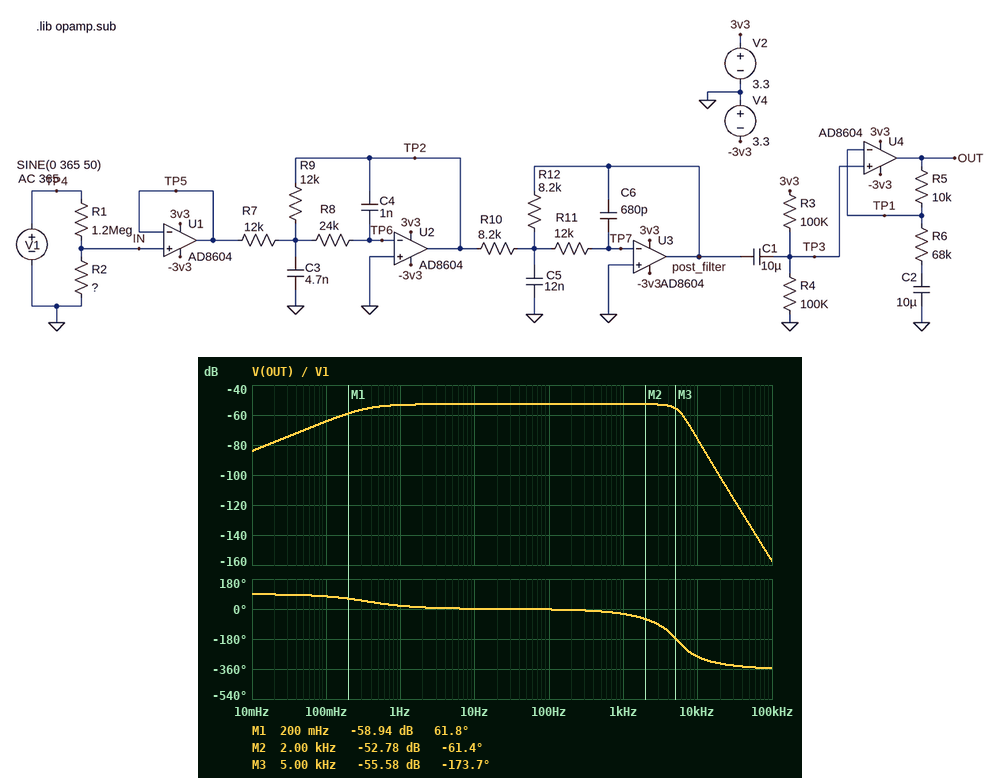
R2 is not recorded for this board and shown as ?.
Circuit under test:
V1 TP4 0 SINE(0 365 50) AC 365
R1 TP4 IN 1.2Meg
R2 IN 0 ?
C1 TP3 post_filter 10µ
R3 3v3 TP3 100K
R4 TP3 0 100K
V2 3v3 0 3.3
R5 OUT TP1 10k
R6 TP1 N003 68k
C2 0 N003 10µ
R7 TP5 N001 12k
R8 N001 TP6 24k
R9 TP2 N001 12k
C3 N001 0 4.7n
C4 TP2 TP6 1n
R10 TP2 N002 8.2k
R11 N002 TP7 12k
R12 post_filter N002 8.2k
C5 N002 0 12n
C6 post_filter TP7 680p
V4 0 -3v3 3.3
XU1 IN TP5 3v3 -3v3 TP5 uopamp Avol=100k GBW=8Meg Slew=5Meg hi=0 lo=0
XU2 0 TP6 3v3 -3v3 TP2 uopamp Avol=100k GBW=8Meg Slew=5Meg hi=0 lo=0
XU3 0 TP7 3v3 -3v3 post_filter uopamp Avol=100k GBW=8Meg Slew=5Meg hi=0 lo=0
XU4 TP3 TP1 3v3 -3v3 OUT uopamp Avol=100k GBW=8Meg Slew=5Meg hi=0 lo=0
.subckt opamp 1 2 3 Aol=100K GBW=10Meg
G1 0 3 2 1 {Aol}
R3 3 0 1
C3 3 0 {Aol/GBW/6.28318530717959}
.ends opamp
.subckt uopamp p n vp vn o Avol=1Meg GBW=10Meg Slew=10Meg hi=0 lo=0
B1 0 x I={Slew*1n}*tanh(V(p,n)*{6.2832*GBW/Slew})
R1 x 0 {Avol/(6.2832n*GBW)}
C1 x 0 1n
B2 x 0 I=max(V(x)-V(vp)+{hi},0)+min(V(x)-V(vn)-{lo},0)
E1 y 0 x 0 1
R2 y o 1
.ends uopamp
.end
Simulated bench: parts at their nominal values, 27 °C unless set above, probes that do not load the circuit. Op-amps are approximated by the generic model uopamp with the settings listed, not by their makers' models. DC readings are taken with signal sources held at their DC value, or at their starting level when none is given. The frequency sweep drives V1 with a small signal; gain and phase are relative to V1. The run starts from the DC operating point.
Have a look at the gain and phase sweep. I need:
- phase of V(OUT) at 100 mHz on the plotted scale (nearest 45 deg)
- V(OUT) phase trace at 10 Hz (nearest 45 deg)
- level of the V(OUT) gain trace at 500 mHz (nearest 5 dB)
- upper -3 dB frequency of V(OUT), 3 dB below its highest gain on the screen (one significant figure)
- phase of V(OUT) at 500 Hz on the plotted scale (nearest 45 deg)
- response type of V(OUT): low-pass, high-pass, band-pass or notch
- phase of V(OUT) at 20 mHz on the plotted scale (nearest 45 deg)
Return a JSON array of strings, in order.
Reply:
["90 deg", "0 deg", "-55 dB", "5 kHz", "0 deg", "band-pass", "90 deg"]
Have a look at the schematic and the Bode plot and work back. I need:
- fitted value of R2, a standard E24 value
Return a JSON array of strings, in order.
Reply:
["2.4 kΩ"]
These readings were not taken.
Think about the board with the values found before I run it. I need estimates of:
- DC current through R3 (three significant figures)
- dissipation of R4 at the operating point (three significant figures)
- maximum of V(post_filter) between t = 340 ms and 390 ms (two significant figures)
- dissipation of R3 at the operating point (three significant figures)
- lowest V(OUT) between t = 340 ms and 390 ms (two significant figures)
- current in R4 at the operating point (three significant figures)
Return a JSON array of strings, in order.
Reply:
["16.5 µA", "27.2 µW", "730 mV", "27.2 µW", "810 mV", "16.5 µA"]
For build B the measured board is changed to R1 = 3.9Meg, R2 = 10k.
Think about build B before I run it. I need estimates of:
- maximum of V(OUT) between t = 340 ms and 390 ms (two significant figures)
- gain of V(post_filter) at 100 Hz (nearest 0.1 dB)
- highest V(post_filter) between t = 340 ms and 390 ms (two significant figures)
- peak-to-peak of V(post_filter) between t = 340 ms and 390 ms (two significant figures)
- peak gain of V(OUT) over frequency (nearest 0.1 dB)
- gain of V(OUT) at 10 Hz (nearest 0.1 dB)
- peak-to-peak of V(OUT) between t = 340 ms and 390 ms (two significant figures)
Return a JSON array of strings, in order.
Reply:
["2.7 V", "-51.8 dB", "930 mV", "1.9 V", "-50.6 dB", "-50.7 dB", "2.1 V"]
